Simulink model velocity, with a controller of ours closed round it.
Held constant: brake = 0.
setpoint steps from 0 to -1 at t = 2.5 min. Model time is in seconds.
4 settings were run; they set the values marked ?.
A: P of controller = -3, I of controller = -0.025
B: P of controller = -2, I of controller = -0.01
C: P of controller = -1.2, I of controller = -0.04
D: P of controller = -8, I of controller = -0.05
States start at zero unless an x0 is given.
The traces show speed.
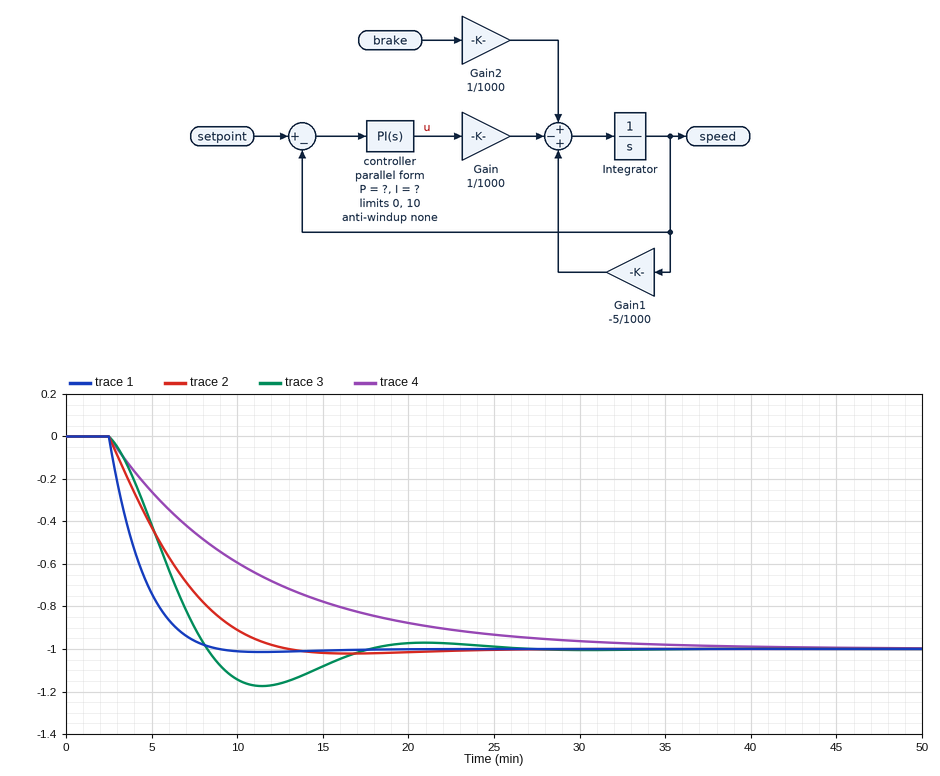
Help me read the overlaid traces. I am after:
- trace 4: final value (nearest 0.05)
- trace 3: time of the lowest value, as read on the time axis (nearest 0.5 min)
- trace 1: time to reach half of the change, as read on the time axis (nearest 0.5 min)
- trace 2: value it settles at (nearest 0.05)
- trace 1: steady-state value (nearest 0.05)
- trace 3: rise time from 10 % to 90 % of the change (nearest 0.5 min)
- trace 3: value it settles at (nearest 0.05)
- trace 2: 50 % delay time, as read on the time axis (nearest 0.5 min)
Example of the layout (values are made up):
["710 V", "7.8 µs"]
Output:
["-1.00", "11.5 min", "4.0 min", "-1.00", "-1.00", "4.0 min", "-1.00", "5.5 min"]
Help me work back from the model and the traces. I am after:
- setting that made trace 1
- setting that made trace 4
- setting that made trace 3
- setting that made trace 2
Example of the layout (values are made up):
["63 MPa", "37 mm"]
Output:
["D", "B", "C", "A"]
